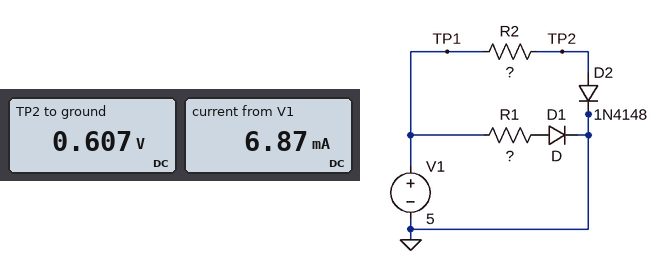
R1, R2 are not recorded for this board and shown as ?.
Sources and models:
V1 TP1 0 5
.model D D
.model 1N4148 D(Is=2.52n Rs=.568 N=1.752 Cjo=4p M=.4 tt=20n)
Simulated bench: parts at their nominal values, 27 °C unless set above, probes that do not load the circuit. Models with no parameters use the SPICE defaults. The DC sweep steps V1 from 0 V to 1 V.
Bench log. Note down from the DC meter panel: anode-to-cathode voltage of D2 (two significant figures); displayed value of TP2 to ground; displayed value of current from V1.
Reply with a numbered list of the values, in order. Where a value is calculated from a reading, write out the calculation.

1. 607 mV = 610 mV
2. 0.607 V
3. 6.87 mA
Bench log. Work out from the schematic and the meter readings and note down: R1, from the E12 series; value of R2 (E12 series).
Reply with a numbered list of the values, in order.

1. 820 Ω
2. 2.7 kΩ
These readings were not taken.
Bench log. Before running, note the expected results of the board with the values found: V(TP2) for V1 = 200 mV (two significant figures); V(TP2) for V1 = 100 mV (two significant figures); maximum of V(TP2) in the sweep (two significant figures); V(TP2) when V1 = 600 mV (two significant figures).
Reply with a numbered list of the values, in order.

1. 200 mV
2. 100 mV
3. 510 mV
4. 450 mV
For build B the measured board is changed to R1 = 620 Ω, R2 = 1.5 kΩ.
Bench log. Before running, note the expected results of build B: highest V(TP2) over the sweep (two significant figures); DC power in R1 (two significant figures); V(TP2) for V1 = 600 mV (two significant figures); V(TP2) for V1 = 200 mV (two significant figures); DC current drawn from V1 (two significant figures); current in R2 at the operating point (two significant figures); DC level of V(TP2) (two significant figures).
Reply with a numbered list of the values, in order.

1. 530 mV
2. 30 mW
3. 470 mV
4. 200 mV
5. 9.8 mA
6. 2.9 mA
7. 630 mV
